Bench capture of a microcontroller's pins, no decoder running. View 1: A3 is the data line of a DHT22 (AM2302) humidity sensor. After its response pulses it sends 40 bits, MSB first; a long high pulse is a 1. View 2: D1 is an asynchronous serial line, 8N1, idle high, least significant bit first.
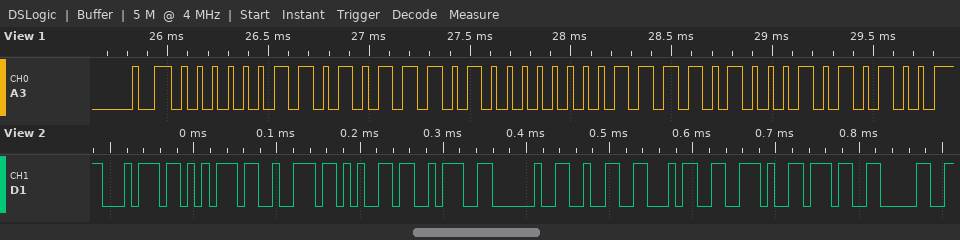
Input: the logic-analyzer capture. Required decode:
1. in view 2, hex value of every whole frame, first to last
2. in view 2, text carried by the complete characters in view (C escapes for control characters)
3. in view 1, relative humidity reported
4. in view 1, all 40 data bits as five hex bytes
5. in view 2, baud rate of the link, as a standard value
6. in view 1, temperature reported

74 75 72 65 3A 20 32 34 2E 37 30
"ture: 24.70"
86.1 %
03 5D 00 F4 54
115200 baud
24.4 °C
